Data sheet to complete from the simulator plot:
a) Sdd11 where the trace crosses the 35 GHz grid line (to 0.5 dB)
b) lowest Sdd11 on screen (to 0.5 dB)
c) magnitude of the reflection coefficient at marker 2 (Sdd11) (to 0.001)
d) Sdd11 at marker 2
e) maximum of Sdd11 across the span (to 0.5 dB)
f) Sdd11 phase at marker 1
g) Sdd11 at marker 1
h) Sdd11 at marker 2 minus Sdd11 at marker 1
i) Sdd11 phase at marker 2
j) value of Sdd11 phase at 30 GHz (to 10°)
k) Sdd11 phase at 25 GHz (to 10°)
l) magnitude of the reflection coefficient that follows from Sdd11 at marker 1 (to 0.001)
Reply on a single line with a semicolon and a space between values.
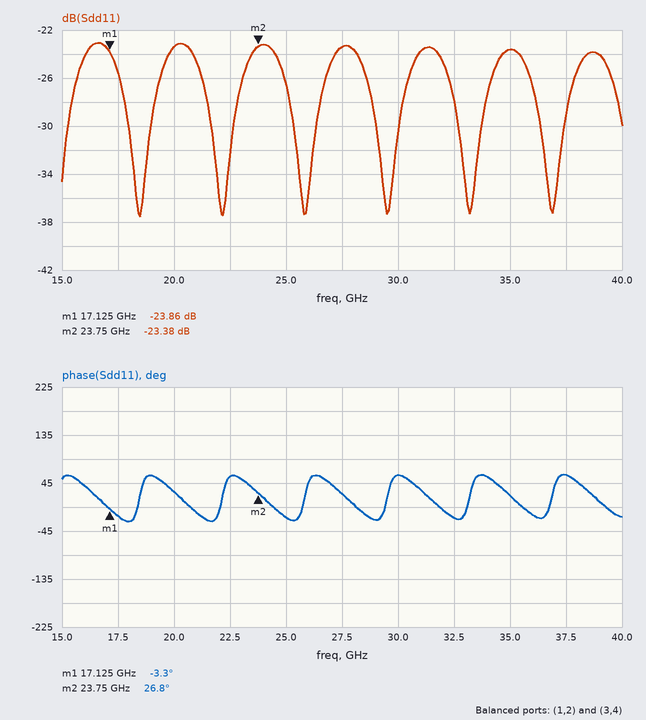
-23.5 dB; -37.5 dB; 0.068; -23.38 dB; -23.0 dB; -3.3°; -23.86 dB; 0.48 dB; 26.8°; 60°; -20°; 0.064
